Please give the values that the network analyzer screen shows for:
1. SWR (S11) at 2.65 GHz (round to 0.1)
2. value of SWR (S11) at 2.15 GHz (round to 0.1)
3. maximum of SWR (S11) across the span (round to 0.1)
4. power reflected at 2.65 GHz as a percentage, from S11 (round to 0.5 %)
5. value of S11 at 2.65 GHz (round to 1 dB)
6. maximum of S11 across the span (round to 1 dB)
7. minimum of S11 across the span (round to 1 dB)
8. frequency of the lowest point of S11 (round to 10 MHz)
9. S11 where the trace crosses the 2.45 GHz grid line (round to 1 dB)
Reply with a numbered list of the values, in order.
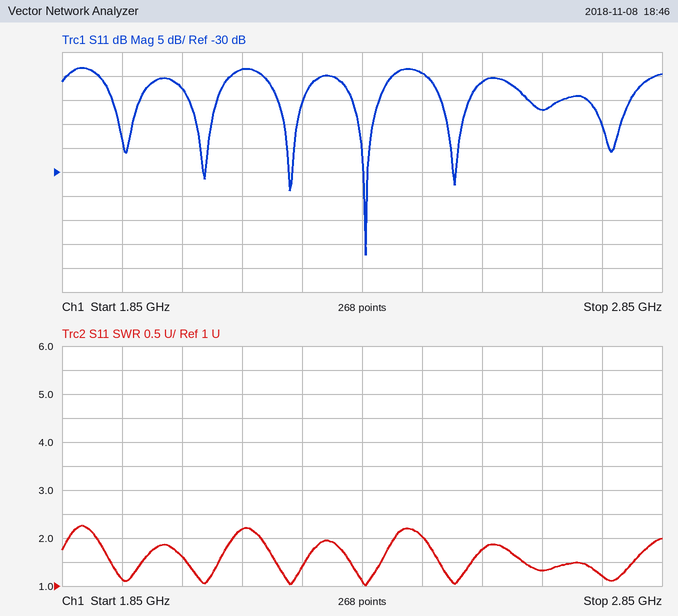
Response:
1. 1.3
2. 2.2
3. 2.3
4. 2.0 %
5. -17 dB
6. -8 dB
7. -47 dB
8. 2.36 GHz
9. -9 dB
